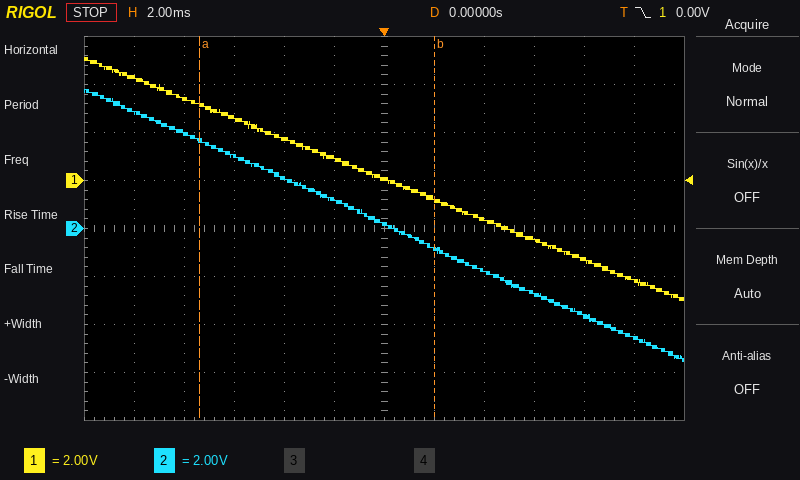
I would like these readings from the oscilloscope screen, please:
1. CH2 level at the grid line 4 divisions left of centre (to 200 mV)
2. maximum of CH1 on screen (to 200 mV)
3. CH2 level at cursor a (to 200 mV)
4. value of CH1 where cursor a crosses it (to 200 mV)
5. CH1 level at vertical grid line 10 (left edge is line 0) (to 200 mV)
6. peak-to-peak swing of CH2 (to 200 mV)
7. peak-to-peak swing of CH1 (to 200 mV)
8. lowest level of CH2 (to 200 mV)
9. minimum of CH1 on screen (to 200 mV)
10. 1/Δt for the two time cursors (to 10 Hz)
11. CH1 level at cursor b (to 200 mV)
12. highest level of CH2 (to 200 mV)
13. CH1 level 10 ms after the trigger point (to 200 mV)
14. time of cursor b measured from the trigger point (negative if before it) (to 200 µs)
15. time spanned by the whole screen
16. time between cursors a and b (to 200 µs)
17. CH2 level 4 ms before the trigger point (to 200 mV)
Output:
4.0 V
5.2 V
3.6 V
3.2 V
-3.4 V
11.4 V
10.2 V
-5.6 V
-5.0 V
110 Hz
-800 mV
5.8 V
-4.2 V
+2.0 ms
24 ms
9.4 ms
2.2 V
